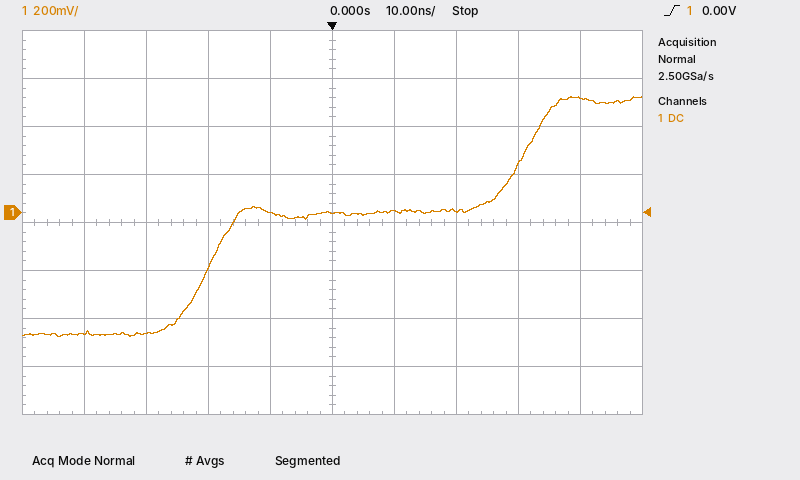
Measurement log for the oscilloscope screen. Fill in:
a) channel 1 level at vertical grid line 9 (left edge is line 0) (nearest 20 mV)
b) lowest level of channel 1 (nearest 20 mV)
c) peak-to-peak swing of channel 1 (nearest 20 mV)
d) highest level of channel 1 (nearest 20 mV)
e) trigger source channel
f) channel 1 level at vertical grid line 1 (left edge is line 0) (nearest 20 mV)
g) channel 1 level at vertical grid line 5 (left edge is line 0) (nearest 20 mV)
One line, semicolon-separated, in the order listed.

480 mV; -520 mV; 1.00 V; 480 mV; channel 1; -500 mV; 0 mV
